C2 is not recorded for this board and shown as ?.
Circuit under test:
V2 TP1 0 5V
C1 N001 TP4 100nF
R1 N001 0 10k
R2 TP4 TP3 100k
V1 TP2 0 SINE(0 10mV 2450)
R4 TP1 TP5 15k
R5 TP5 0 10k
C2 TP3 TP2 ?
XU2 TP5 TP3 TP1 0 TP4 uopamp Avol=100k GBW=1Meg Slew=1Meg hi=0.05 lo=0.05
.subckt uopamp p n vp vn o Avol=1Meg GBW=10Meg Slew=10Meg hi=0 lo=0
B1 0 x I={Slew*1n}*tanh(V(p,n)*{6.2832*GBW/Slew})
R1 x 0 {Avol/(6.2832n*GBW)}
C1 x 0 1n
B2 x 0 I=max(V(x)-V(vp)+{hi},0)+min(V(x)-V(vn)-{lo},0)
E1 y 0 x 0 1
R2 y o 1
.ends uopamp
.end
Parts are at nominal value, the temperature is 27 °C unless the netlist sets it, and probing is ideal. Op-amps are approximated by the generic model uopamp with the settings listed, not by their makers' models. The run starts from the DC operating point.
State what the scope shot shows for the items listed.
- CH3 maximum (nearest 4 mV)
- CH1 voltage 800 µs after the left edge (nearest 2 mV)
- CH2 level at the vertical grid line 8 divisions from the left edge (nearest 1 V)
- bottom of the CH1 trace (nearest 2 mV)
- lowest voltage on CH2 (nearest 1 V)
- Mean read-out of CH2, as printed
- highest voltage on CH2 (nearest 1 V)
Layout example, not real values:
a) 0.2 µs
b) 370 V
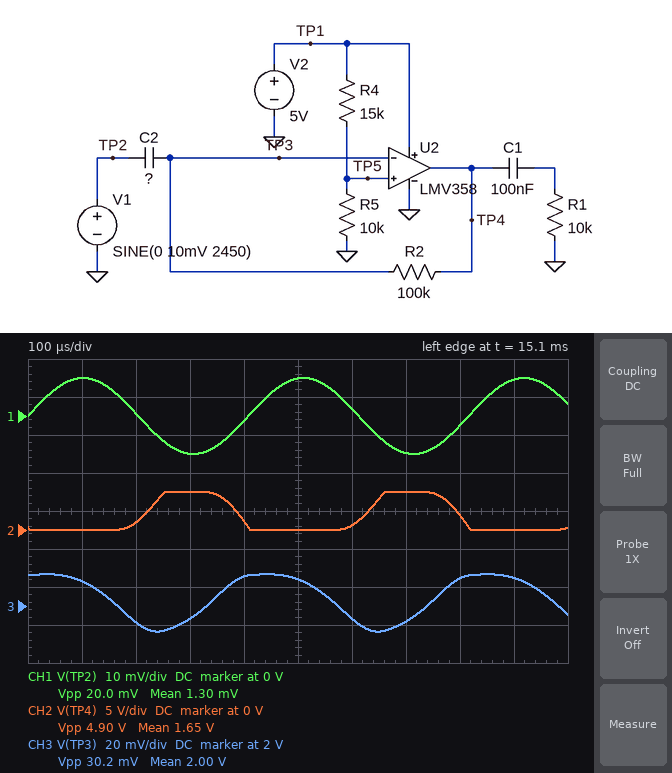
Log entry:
a) 2.016 V
b) -2 mV
c) 2 V
d) -10 mV
e) 0 V
f) 1.65 V
g) 5 V
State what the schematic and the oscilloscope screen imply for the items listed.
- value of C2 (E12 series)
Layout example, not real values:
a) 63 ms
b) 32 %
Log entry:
a) 150 nF
